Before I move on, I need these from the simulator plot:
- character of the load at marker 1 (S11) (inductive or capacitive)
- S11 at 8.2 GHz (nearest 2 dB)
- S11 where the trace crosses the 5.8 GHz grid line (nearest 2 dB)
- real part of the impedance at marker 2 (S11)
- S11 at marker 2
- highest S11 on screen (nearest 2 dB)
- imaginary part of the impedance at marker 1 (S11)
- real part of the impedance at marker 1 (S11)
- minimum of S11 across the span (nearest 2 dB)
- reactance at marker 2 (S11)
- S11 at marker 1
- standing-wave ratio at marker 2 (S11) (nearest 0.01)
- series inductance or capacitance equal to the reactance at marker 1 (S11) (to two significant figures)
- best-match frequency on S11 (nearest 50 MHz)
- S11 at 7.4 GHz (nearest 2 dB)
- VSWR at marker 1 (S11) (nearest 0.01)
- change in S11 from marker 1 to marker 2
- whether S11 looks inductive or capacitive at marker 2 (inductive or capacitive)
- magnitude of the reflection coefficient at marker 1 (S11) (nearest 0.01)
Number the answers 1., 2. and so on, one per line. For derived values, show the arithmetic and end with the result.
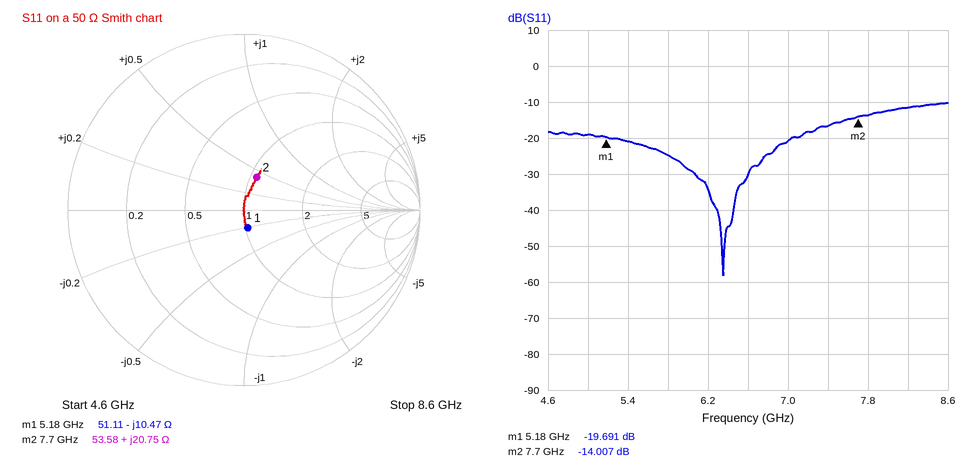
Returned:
1. capacitive
2. -12 dB
3. -24 dB
4. 53.58 Ω
5. -14.007 dB
6. -10 dB
7. -10.47 Ω
8. 51.11 Ω
9. -58 dB
10. +20.75 Ω
11. -19.691 dB
12. 1.50
13. C = 1/(2π × 5.18 GHz × 10.47 Ω) ≈ 2.9 pF
14. 6.35 GHz
15. -16 dB
16. (1 + 0.1036)/(1 − 0.1036) ≈ 1.23
17. -14.007 − (-19.691) = 5.684 dB
18. inductive
19. 0.10
